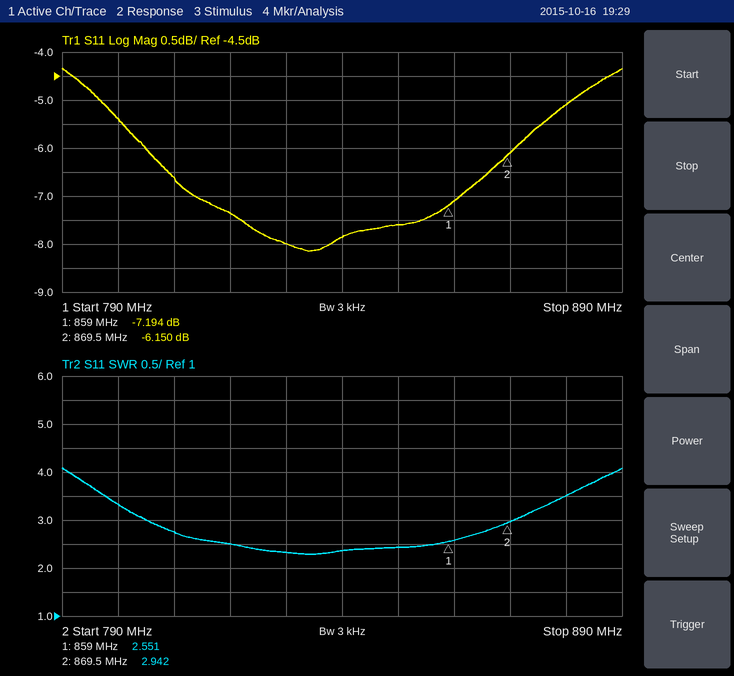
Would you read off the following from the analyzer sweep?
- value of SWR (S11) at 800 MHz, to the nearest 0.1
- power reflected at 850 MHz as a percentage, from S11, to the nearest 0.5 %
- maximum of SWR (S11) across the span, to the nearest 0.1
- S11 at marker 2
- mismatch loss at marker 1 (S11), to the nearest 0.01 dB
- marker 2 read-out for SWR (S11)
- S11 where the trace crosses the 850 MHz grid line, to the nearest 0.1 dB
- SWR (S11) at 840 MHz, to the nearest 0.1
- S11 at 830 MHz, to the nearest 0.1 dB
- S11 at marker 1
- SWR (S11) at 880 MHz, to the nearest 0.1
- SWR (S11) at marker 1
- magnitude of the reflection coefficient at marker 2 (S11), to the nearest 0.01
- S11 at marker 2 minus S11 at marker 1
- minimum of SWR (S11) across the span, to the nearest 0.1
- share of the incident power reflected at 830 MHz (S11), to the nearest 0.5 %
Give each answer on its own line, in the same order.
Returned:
3.3
17.5 %
4.1
-6.150 dB
0.92 dB
2.942
-7.6 dB
2.4
-8.0 dB
-7.194 dB
3.5
2.551
0.49
1.044 dB
2.3
16.0 %
